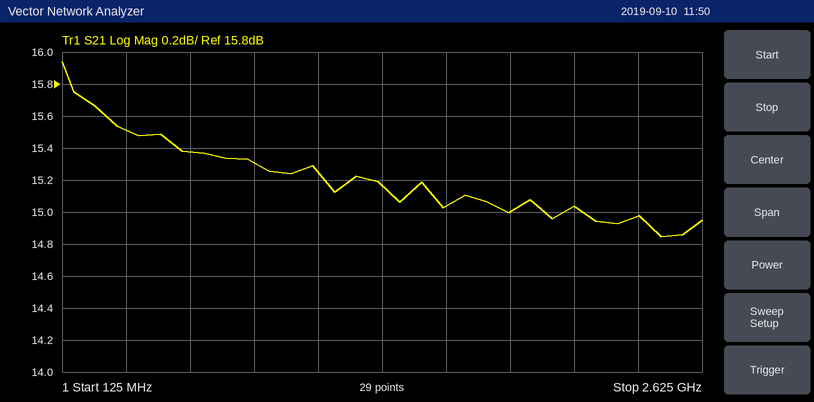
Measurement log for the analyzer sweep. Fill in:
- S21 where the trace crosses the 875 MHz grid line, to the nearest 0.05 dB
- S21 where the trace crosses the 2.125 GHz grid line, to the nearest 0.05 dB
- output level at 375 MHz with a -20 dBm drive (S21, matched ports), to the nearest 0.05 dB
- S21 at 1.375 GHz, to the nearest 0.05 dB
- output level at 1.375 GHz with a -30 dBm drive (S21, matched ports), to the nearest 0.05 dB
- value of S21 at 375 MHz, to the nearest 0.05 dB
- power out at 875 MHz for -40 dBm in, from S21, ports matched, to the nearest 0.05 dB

15.30 dB
15.05 dB
-4.50 dBm
15.15 dB
-14.85 dBm
15.50 dB
-24.70 dBm
